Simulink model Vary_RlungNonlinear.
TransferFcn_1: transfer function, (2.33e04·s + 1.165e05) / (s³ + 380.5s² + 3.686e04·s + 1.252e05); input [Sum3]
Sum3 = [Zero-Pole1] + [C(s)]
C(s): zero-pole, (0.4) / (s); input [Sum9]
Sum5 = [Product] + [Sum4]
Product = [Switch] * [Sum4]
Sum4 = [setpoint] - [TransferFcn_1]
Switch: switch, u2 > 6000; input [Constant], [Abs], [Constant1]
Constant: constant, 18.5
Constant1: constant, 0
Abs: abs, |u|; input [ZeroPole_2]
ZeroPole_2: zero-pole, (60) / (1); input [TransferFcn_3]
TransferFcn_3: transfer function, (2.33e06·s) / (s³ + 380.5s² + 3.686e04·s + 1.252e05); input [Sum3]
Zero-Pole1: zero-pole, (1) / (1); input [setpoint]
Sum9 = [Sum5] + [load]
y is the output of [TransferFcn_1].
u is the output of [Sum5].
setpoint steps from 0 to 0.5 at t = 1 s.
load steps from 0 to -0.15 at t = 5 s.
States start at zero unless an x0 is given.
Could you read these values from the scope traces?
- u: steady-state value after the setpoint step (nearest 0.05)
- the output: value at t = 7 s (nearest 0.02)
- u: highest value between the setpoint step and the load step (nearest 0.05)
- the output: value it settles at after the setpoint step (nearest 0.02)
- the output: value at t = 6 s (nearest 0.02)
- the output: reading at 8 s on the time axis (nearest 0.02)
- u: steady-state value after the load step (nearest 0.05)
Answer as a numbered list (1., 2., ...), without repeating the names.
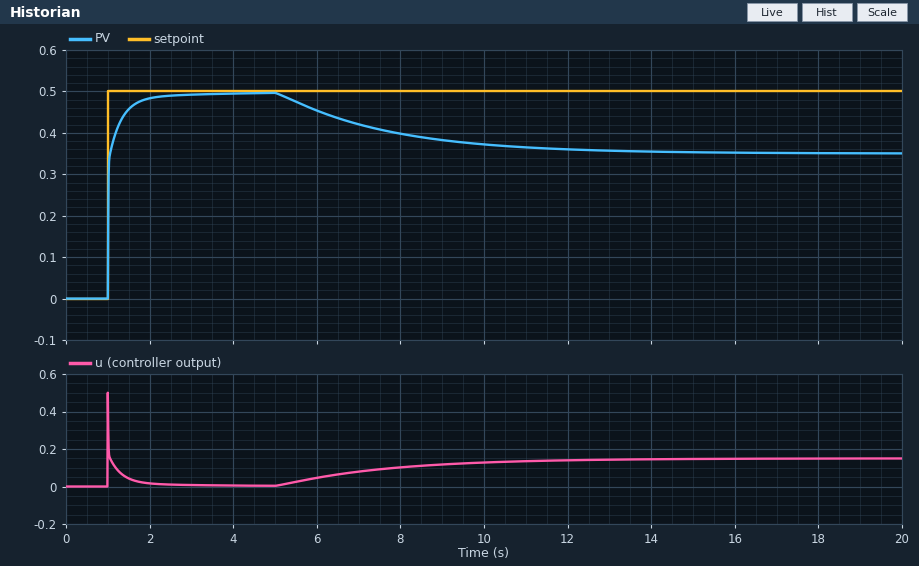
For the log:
1. 0.00
2. 0.42
3. 0.50
4. 0.50
5. 0.46
6. 0.40
7. 0.15
